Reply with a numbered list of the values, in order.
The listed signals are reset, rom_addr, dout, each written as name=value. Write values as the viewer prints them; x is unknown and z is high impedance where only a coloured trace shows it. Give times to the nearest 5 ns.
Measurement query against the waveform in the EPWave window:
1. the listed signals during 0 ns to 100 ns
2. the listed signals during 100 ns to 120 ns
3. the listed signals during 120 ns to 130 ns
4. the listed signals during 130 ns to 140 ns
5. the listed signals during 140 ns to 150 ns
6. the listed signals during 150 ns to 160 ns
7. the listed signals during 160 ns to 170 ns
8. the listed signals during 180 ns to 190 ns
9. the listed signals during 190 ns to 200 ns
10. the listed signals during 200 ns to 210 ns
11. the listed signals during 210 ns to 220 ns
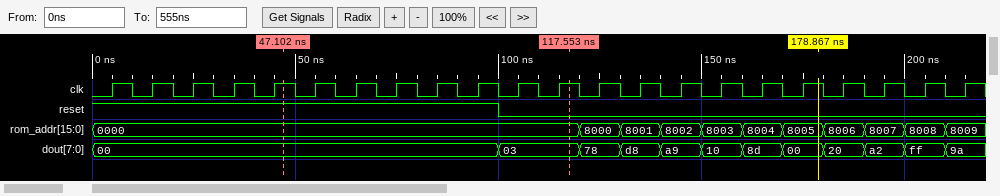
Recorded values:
1. reset=1, rom_addr=0000, dout=00
2. reset=0, rom_addr=0000, dout=03
3. reset=0, rom_addr=8000, dout=78
4. reset=0, rom_addr=8001, dout=d8
5. reset=0, rom_addr=8002, dout=a9
6. reset=0, rom_addr=8003, dout=10
7. reset=0, rom_addr=8004, dout=8d
8. reset=0, rom_addr=8006, dout=20
9. reset=0, rom_addr=8007, dout=a2
10. reset=0, rom_addr=8008, dout=ff
11. reset=0, rom_addr=8009, dout=9a
